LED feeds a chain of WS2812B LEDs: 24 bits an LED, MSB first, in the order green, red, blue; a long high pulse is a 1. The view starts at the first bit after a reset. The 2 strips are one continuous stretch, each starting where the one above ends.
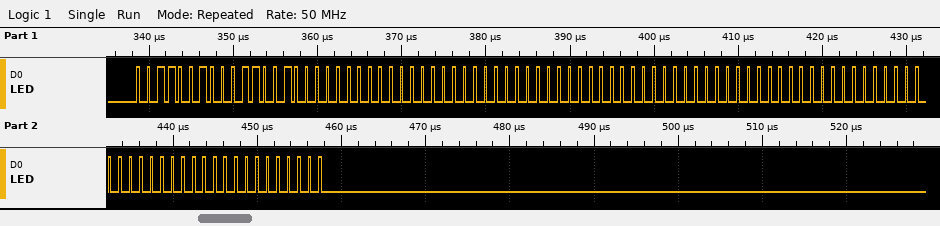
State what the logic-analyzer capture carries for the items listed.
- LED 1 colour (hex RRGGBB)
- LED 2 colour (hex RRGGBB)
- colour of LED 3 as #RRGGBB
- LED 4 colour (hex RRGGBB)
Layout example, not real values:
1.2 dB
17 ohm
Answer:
#323200
#000000
#000000
#000000
